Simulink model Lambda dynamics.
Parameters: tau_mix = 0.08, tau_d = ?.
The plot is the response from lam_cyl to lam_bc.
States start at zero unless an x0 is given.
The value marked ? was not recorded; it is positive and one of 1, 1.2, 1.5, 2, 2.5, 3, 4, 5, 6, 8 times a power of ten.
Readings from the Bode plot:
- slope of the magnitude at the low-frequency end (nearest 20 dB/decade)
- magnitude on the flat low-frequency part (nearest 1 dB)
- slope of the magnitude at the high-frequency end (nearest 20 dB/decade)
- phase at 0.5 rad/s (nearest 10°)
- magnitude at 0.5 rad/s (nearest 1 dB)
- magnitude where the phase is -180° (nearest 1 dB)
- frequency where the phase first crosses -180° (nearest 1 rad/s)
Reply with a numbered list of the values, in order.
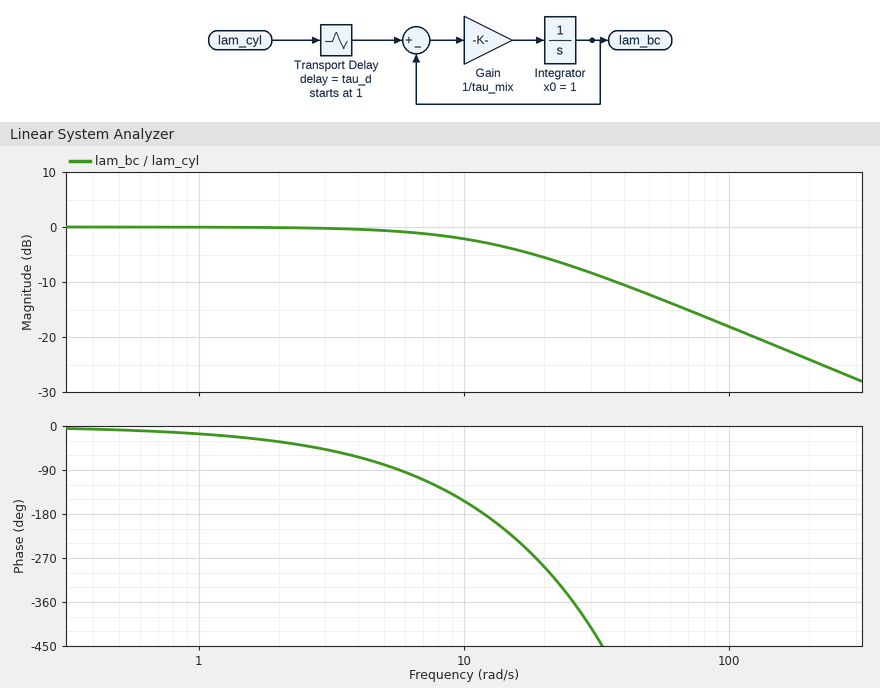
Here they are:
1. 0 dB/decade
2. 0 dB
3. -20 dB/decade
4. -10°
5. 0 dB
6. -3 dB
7. 12 rad/s
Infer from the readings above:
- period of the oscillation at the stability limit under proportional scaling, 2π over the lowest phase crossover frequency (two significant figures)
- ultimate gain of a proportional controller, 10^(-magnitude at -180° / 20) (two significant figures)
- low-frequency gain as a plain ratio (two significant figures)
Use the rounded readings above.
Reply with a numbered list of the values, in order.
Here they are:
1. 0.52 s
2. 1.4
3. 1.0
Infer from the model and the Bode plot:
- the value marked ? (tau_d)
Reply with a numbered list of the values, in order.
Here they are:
1. 0.2
